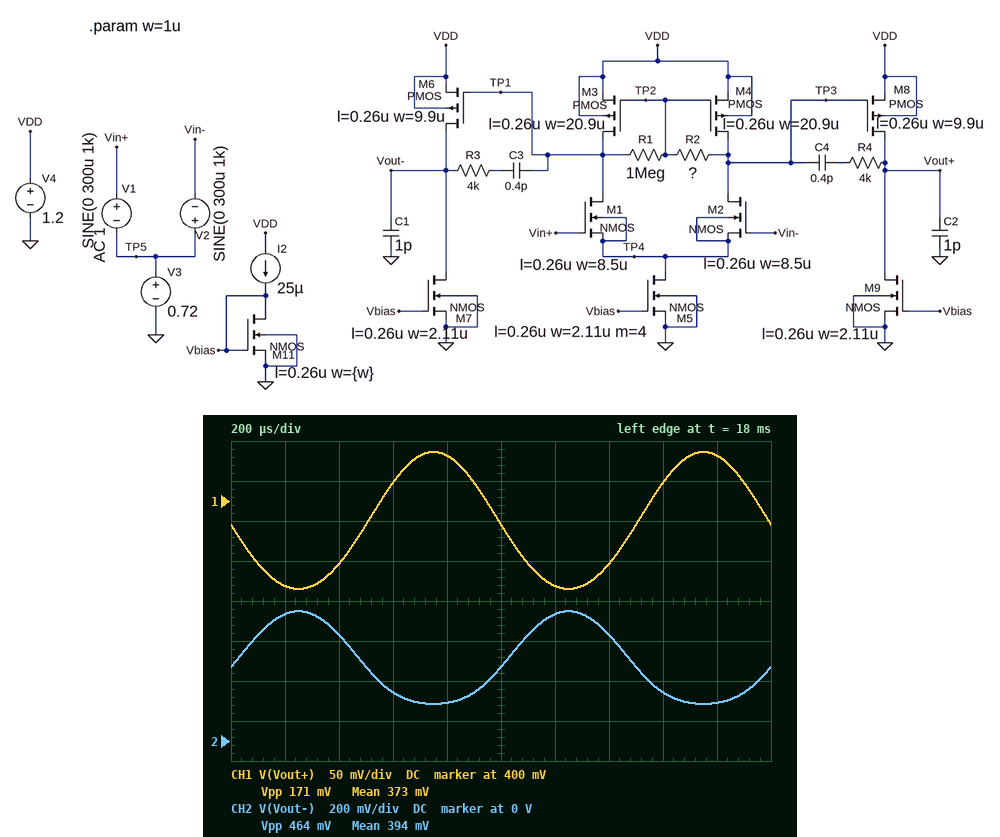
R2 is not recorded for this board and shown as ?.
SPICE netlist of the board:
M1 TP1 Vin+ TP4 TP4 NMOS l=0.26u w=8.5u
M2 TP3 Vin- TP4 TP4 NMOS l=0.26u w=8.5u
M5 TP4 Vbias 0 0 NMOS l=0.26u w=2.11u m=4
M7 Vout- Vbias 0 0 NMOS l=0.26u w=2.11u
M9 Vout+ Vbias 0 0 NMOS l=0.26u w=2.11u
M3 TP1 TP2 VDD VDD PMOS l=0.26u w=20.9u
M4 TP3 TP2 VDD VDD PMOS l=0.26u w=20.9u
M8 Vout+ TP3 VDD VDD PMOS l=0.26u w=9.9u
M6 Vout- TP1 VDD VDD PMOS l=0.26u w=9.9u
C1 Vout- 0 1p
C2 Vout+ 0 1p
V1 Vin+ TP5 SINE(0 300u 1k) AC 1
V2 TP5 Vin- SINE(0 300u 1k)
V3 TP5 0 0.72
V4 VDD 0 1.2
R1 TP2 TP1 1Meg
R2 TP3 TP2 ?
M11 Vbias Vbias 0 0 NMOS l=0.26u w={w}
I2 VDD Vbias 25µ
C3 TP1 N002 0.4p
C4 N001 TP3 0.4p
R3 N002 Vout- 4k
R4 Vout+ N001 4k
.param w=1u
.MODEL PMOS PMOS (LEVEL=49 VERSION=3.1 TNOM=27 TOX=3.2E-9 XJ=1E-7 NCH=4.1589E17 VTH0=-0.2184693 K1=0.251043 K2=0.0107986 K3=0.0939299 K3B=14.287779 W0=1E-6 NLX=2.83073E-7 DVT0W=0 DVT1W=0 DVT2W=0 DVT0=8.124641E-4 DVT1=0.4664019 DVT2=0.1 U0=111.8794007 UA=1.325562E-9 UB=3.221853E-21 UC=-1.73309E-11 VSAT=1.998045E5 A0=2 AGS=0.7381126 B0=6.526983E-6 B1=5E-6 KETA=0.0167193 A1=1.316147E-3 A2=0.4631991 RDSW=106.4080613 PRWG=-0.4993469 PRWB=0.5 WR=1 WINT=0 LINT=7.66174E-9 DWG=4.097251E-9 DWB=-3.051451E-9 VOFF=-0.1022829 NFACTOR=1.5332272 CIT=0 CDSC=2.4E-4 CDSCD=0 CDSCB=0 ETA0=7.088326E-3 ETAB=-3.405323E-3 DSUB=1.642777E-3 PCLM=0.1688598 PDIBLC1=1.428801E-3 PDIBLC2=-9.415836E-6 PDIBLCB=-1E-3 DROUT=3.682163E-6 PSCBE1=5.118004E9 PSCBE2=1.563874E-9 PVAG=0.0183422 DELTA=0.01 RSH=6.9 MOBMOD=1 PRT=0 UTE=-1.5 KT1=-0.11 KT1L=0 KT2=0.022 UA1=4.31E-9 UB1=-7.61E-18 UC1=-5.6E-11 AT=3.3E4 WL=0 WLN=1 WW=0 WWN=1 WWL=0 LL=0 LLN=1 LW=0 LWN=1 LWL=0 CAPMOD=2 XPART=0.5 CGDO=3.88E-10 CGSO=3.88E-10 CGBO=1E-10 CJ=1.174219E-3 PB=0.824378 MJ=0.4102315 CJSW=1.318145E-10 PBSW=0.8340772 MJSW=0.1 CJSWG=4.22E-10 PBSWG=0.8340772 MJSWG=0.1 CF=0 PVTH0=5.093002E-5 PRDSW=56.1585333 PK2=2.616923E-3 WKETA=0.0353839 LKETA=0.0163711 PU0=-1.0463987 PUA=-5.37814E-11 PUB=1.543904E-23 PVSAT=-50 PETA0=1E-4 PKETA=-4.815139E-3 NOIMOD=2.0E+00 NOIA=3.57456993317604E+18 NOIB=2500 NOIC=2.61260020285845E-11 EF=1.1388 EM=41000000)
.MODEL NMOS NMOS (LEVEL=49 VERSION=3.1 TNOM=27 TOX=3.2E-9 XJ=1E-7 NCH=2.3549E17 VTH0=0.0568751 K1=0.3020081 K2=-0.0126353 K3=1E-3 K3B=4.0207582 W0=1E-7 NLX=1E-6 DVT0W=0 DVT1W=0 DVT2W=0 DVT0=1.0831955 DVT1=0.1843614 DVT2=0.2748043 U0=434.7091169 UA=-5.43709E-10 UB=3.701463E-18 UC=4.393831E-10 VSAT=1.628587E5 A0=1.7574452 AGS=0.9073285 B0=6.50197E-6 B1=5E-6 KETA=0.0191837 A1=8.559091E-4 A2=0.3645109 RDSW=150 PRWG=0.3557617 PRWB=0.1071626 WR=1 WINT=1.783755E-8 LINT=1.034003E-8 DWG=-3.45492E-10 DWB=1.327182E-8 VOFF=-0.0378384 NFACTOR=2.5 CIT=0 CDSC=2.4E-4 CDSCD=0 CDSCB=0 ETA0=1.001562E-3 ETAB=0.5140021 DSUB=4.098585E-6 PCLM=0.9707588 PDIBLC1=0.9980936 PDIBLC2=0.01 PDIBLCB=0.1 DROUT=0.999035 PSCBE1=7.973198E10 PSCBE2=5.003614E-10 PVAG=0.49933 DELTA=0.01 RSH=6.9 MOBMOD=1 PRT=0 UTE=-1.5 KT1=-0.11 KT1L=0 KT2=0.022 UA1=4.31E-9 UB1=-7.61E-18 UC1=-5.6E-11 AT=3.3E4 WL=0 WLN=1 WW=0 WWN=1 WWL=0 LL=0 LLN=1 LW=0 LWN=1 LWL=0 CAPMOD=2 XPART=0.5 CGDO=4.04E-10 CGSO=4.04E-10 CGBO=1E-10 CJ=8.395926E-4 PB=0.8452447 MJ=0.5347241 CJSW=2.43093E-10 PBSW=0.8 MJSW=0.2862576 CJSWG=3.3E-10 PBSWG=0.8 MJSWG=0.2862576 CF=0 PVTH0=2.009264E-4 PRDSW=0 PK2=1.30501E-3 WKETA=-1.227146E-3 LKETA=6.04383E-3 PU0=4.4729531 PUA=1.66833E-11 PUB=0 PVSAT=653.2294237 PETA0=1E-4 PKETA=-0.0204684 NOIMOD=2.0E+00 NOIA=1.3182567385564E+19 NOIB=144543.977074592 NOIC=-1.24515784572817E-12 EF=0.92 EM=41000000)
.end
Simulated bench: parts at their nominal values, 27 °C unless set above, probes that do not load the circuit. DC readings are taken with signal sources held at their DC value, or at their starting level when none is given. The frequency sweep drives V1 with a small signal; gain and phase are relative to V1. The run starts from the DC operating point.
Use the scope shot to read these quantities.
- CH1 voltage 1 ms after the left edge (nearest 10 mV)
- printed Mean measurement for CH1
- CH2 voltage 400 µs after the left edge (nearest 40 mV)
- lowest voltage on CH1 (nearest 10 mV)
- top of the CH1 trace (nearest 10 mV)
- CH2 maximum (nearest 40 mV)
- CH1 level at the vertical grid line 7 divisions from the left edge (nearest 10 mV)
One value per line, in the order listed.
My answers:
370 mV
373 mV
520 mV
290 mV
460 mV
640 mV
320 mV
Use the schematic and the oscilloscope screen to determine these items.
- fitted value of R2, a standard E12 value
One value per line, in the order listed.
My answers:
330 kΩ
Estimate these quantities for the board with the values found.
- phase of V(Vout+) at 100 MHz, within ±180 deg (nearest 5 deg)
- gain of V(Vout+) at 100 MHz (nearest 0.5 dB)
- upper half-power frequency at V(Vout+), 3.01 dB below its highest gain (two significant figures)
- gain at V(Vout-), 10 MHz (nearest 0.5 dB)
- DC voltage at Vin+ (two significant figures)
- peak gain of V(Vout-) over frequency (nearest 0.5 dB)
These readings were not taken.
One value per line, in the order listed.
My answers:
70 deg
5.0 dB
830 kHz
30.0 dB
720 mV
52.5 dB
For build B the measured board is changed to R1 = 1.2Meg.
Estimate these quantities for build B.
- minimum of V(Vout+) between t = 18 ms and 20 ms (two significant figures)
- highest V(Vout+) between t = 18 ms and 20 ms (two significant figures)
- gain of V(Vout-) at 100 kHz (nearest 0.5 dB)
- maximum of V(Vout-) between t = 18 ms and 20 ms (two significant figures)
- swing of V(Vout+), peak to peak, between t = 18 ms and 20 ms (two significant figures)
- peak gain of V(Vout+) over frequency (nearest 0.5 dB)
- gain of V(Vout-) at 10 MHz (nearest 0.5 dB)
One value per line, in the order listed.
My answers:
300 mV
450 mV
53.0 dB
660 mV
150 mV
42.0 dB
30.5 dB
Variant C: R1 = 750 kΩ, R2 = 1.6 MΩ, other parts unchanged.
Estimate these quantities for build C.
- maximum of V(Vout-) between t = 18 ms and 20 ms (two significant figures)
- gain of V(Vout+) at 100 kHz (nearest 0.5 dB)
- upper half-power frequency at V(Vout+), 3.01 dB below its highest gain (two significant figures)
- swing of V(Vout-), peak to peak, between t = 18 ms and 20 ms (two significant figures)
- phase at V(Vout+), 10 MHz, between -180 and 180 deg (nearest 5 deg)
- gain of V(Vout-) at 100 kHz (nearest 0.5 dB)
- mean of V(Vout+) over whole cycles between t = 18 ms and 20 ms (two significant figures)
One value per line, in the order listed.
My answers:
490 mV
51.5 dB
810 kHz
220 mV
80 deg
45.5 dB
390 mV
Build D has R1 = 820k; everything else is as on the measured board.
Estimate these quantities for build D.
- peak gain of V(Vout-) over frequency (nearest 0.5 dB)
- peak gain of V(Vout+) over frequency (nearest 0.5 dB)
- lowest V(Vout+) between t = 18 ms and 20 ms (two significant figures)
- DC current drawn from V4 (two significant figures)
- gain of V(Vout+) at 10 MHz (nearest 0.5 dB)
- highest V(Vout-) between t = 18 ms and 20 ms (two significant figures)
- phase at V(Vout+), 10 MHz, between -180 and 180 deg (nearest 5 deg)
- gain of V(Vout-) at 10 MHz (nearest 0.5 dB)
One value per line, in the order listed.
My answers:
52.0 dB
44.5 dB
280 mV
330 µA
24.0 dB
630 mV
105 deg
29.5 dB
